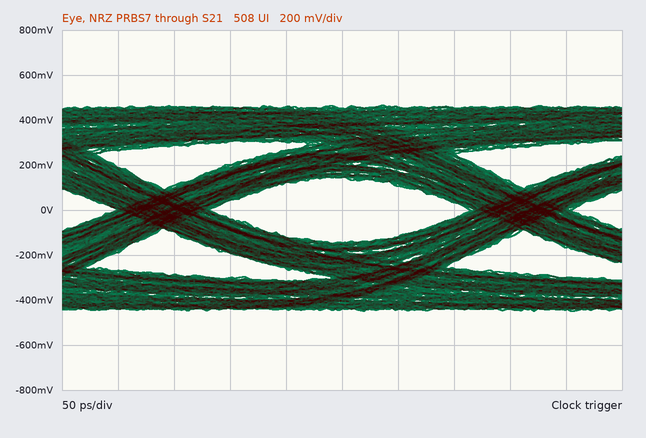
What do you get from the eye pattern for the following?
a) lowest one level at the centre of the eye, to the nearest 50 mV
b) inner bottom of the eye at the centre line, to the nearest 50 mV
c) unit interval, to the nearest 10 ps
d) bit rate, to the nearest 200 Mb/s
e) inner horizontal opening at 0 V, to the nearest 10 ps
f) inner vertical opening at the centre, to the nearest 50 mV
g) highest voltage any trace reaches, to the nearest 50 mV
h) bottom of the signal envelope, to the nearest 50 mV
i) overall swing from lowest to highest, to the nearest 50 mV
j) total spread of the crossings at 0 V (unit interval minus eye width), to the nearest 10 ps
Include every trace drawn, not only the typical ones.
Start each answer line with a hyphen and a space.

- 150 mV
- -150 mV
- 320 ps
- 3.2 Gb/s
- 230 ps
- 300 mV
- 450 mV
- -450 mV
- 900 mV
- 90 ps
